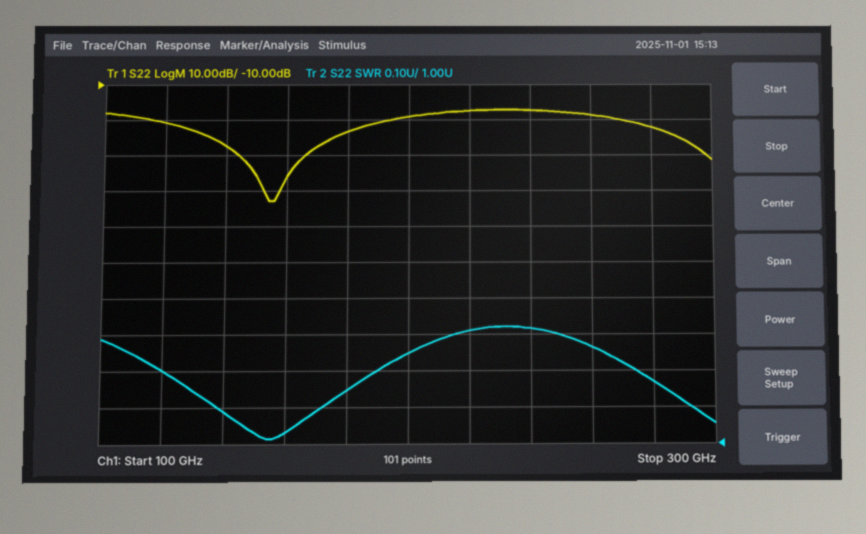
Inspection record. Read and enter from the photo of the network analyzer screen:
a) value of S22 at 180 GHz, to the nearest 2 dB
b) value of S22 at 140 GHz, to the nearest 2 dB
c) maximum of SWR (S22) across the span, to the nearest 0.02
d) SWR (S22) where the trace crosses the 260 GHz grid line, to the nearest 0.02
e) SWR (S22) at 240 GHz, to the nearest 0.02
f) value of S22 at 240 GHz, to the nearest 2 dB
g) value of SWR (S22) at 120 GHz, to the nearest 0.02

-24 dB
-28 dB
1.32
1.26
1.32
-18 dB
1.20
